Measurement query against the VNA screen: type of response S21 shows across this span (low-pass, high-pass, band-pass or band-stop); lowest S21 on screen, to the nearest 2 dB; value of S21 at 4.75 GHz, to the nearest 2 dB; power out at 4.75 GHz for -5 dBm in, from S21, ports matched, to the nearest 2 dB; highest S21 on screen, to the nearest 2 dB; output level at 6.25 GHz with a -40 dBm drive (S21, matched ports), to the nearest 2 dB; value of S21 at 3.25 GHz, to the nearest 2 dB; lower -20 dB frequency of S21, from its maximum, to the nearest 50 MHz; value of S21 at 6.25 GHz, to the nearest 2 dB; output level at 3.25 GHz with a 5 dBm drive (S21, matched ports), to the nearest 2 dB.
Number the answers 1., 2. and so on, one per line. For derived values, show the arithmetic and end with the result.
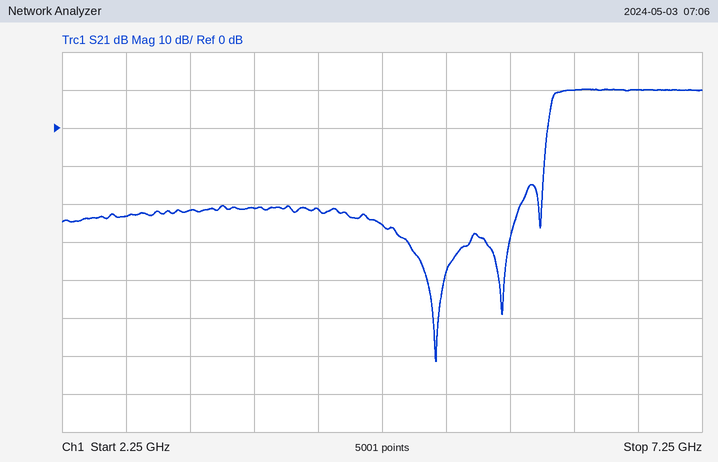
1. high-pass
2. -62 dB
3. -26 dB
4. -5 dBm + (-26 dB) = -30 dBm
5. 10 dB
6. -40 dBm + (10 dB) = -30 dBm
7. -22 dB
8. 6.00 GHz
9. 10 dB
10. 5 dBm + (-22 dB) = -16 dBm
